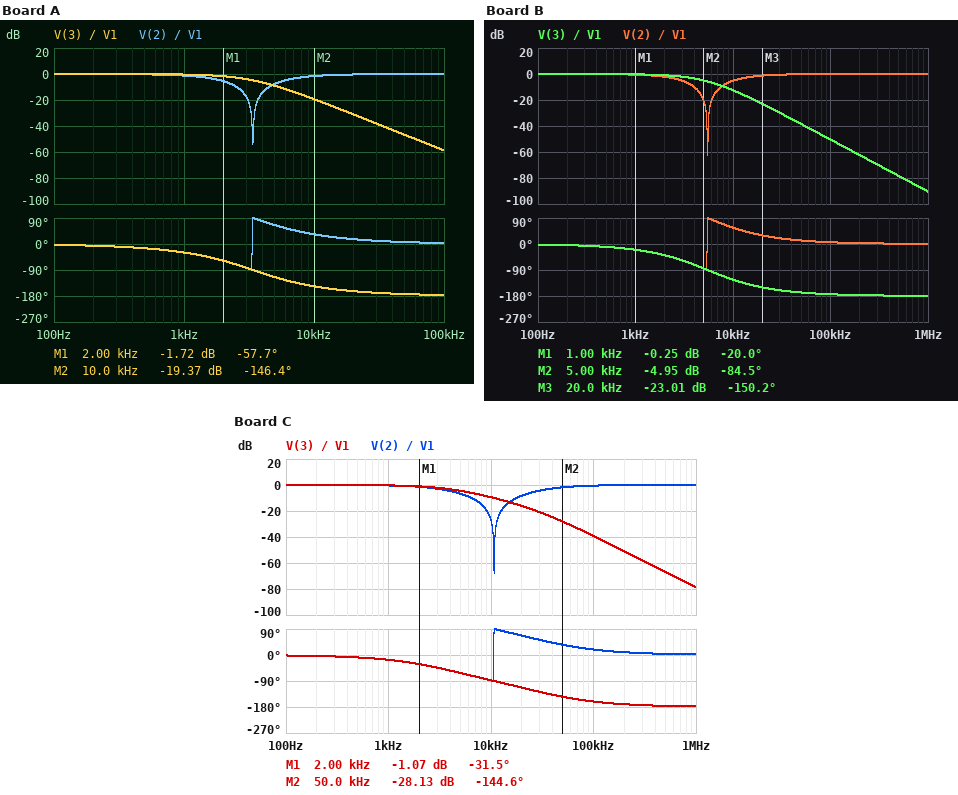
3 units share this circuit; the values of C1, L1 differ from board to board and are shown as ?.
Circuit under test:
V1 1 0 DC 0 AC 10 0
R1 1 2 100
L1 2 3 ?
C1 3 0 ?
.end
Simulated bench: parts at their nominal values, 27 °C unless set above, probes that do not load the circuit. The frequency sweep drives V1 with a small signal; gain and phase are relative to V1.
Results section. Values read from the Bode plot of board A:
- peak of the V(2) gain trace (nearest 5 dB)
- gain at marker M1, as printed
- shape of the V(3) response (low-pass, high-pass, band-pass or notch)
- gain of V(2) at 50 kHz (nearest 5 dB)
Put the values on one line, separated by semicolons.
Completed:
0 dB; -1.72 dB; low-pass; 0 dB
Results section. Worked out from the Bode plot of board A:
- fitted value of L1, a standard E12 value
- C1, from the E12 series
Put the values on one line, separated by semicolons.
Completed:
2.7 mH; 820 nF
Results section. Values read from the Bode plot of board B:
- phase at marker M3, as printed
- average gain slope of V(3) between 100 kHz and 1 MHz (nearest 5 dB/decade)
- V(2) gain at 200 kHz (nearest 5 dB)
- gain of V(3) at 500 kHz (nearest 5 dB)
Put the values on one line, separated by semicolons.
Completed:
-150.2 deg; -40 dB/decade; 0 dB; -80 dB
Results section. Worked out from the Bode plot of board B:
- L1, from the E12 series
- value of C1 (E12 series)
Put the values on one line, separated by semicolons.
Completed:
1.5 mH; 560 nF
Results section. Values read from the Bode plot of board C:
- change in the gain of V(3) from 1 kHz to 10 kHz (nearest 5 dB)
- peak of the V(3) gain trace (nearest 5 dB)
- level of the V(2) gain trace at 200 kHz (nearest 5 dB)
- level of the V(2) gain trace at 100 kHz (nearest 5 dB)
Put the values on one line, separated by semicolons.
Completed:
-10 dB; 0 dB; 0 dB; 0 dB
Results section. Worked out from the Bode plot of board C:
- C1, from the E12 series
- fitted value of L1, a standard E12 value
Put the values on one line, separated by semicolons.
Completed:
470 nF; 470 µH
